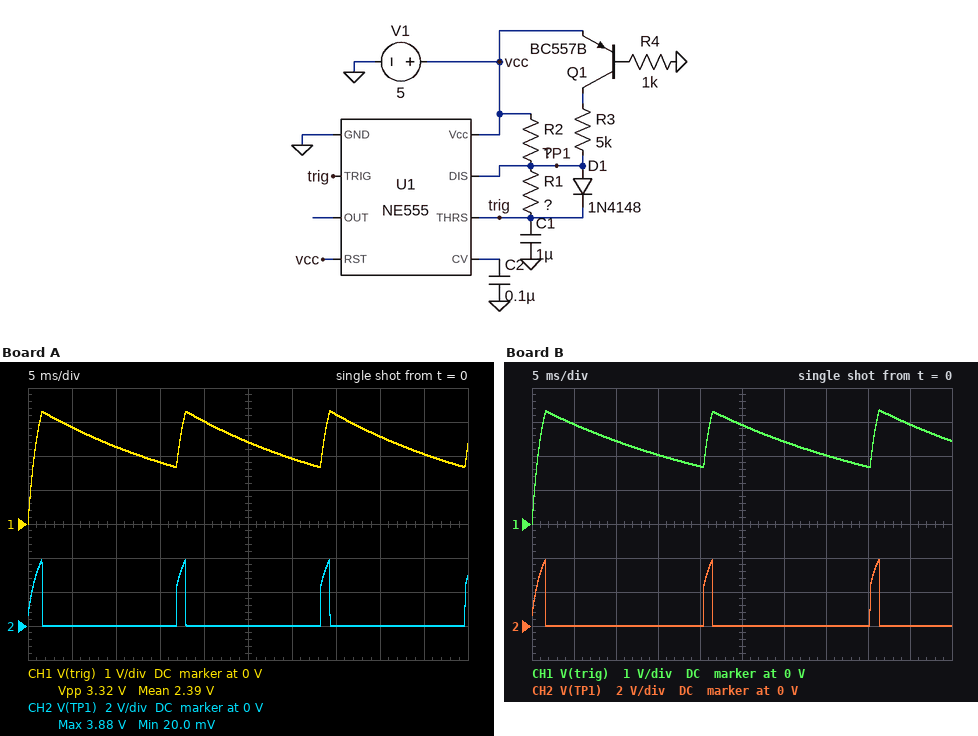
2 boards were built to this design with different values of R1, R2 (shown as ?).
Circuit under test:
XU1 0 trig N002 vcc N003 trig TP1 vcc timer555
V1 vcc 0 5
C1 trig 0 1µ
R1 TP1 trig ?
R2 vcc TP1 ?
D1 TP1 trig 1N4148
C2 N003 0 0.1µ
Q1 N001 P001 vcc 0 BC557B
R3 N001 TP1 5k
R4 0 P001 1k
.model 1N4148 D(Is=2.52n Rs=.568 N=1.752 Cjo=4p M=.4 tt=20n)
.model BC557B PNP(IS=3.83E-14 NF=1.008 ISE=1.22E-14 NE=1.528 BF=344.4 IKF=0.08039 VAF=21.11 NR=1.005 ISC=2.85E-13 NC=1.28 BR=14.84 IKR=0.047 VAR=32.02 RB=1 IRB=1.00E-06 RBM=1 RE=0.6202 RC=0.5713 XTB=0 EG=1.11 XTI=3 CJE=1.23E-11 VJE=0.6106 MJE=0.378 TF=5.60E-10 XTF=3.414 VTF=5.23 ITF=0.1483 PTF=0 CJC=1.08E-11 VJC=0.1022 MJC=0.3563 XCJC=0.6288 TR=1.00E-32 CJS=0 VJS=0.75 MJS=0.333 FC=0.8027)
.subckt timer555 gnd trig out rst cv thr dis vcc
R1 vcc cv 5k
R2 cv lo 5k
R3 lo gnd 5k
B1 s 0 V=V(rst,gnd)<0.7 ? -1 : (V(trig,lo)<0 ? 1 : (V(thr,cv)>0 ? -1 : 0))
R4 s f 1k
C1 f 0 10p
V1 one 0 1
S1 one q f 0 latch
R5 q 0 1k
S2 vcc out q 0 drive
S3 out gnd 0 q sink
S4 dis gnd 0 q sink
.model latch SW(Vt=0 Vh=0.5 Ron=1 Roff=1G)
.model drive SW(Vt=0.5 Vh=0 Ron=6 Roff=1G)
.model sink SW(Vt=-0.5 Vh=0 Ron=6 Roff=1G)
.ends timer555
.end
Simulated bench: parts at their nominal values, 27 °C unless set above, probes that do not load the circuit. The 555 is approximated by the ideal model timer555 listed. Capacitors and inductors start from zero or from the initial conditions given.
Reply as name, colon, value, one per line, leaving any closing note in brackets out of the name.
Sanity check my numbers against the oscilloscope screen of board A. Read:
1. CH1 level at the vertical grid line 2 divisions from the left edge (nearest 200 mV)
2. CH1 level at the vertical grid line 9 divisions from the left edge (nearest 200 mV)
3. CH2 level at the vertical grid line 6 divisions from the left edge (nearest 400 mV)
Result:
CH1 level at the vertical grid line 2 divisions from the left edge: 2.2 V
CH1 level at the vertical grid line 9 divisions from the left edge: 2.0 V
CH2 level at the vertical grid line 6 divisions from the left edge: 0 V
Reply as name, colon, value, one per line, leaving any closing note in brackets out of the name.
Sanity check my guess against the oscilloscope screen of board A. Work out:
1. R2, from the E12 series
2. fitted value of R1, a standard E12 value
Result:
R2, from the E12 series: 1.5 kΩ
fitted value of R1, a standard E12 value: 22 kΩ
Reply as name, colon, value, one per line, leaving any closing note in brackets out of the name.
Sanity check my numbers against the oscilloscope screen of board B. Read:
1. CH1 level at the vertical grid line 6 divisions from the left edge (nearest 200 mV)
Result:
CH1 level at the vertical grid line 6 divisions from the left edge: 2.4 V
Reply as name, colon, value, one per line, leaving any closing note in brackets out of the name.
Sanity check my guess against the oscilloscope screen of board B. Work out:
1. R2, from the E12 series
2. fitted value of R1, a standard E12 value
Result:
R2, from the E12 series: 1.5 kΩ
fitted value of R1, a standard E12 value: 27 kΩ
